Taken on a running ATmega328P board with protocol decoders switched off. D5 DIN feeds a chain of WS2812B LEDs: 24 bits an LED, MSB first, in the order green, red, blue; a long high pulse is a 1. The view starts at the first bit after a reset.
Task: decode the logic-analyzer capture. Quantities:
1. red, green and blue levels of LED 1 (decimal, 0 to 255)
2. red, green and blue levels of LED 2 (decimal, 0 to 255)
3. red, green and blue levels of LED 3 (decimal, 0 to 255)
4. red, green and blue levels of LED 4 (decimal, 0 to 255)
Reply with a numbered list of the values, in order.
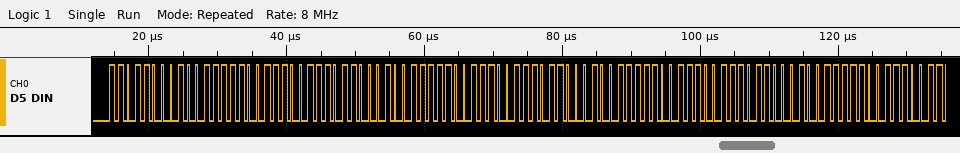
1. 159, 216, 57
2. 159, 216, 57
3. 159, 216, 57
4. 159, 216, 57
